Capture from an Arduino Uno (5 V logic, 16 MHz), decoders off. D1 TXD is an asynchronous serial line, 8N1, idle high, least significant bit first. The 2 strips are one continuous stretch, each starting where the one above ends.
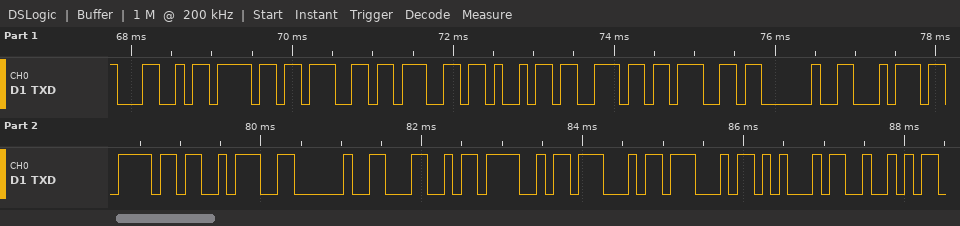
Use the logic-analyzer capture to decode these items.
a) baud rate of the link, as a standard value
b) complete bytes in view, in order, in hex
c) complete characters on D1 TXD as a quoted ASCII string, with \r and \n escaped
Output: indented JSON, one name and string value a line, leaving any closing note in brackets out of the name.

{
  "baud rate of the link, as a standard value": "9600 baud",
  "complete bytes in view, in order, in hex": "4C 6F 67 67 69 6E 67 20 74 6F 3A 20 4C 4F 47 47 45 52",
  "complete characters on D1 TXD as a quoted ASCII string, with \\r and \\n escaped": "\"Logging to: LOGGER\""
}
